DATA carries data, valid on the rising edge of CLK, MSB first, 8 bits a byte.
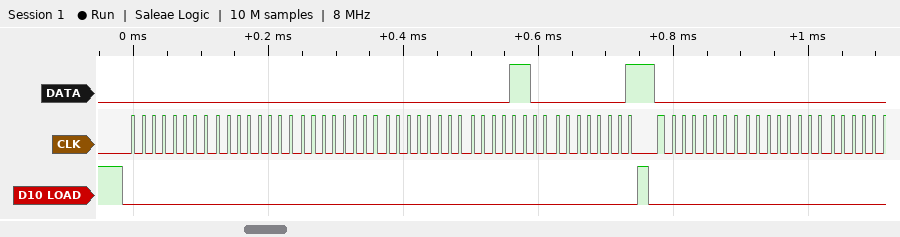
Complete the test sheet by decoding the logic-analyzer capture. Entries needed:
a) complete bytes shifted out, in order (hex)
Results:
0x00 0x00 0x00 0x00 0x0C 0x01 0x00 0x00
